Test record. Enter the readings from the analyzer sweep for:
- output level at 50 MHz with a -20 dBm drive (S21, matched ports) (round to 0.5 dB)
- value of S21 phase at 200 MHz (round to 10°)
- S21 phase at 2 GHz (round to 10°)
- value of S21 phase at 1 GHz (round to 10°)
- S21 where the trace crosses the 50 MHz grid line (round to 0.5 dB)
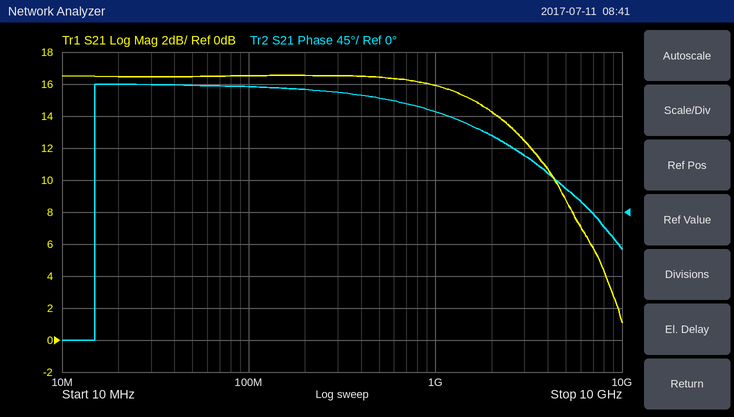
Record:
-3.5 dBm
170°
110°
140°
16.5 dB
